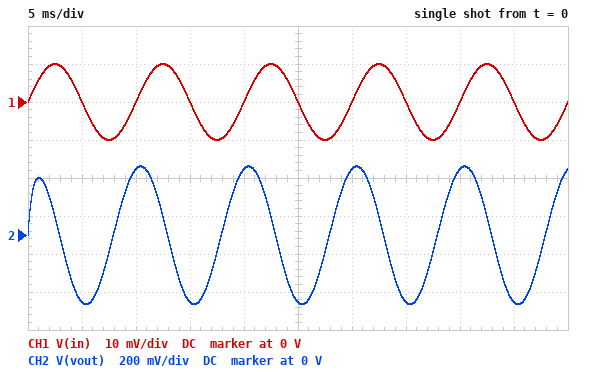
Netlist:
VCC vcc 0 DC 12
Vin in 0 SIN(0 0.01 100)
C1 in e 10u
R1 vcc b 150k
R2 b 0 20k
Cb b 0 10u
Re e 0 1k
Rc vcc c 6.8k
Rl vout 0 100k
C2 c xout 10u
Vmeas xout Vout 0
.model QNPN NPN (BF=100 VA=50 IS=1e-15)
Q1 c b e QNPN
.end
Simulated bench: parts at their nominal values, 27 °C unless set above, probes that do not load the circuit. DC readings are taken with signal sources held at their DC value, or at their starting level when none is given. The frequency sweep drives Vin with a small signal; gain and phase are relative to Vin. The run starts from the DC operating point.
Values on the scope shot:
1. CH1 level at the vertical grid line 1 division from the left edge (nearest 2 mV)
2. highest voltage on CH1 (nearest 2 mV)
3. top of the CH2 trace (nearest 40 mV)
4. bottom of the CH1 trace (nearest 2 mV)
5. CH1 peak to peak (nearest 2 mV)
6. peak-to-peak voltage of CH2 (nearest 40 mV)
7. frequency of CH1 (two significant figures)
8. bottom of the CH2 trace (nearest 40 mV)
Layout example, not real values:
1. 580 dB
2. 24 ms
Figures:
1. 0 V
2. 10 mV
3. 360 mV
4. -10 mV
5. 20 mV
6. 720 mV
7. 100 Hz
8. -360 mV
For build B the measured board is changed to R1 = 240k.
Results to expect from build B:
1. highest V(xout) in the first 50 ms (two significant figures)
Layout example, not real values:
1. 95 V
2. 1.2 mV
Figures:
1. 280 mV
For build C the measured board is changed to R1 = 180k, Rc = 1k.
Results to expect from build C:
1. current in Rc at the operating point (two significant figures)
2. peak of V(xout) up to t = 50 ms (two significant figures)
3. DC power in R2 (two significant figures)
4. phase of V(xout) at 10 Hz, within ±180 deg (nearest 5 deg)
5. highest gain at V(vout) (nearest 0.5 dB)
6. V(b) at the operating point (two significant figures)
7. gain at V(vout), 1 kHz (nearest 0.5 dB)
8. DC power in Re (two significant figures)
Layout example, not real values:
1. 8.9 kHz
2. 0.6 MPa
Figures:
1. 440 µA
2. 54 mV
3. 64 µW
4. 90 deg
5. 24.5 dB
6. 1.1 V
7. 24.0 dB
8. 200 µW
